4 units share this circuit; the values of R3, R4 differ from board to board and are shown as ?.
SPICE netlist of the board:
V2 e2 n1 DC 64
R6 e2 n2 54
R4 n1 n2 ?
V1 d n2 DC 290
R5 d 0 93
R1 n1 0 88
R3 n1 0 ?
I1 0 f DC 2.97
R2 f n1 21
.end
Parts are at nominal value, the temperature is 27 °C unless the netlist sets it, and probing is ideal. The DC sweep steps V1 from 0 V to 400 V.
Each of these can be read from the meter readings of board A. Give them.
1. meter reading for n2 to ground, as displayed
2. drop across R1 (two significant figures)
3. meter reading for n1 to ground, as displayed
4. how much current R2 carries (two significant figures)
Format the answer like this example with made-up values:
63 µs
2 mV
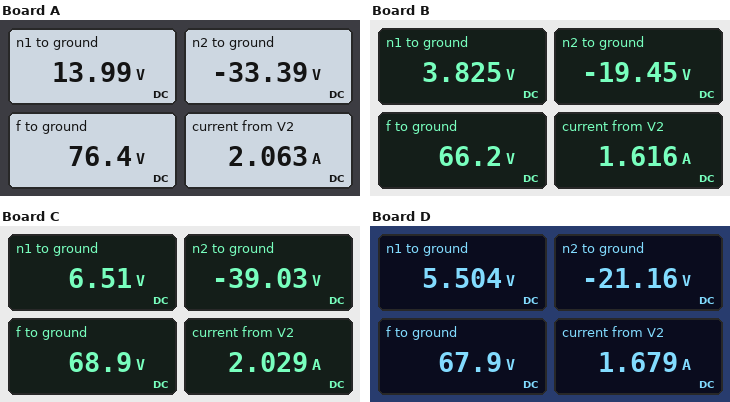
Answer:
-33.39 V
14 V
13.99 V
3.0 A
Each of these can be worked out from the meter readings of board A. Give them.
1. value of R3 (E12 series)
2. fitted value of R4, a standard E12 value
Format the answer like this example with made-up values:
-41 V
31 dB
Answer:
270 Ω
68 Ω
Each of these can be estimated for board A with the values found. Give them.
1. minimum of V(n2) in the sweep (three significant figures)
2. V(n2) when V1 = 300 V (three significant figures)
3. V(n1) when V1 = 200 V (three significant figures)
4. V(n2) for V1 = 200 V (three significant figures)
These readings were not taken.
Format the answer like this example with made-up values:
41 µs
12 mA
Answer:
-89.4 V
-38.5 V
45.5 V
12.4 V
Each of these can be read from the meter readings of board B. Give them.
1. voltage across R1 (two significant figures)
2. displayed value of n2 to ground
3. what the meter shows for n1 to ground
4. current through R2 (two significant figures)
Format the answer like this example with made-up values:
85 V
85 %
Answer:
3.8 V
-19.45 V
3.825 V
3.0 A
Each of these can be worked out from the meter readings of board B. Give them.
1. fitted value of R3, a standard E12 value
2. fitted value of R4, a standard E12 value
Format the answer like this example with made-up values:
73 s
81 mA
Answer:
220 Ω
18 Ω
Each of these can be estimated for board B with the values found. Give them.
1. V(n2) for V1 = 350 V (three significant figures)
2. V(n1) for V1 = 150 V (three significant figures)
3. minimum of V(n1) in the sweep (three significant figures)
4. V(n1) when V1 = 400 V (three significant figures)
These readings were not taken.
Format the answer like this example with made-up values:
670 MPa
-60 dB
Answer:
-46.5 V
55.8 V
-37.0 V
-37.0 V
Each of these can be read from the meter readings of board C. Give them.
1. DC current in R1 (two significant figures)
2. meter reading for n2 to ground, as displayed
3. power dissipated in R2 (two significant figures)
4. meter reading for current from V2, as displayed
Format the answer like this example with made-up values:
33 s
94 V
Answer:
74 mA
-39.03 V
190 W
2.029 A
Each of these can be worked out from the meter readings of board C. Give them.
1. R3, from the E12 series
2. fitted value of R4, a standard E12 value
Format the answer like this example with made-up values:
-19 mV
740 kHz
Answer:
33 Ω
68 Ω
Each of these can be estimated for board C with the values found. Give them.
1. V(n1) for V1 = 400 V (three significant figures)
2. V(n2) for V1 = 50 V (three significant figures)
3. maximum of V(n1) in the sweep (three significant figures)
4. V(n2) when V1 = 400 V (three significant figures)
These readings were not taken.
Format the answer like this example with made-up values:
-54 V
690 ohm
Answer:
-11.4 V
49.2 V
53.8 V
-79.5 V
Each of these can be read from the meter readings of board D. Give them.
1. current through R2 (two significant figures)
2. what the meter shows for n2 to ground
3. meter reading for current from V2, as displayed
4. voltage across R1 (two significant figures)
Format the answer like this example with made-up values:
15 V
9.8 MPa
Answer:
3.0 A
-21.16 V
1.679 A
5.5 V
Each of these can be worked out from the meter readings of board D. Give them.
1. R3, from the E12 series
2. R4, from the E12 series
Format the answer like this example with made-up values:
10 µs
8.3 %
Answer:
330 Ω
22 Ω
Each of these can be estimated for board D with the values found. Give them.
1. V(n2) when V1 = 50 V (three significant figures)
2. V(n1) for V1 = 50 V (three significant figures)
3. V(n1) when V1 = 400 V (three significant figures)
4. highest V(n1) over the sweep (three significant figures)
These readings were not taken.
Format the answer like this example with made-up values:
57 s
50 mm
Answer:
93.5 V
99.1 V
-37.4 V
119 V
